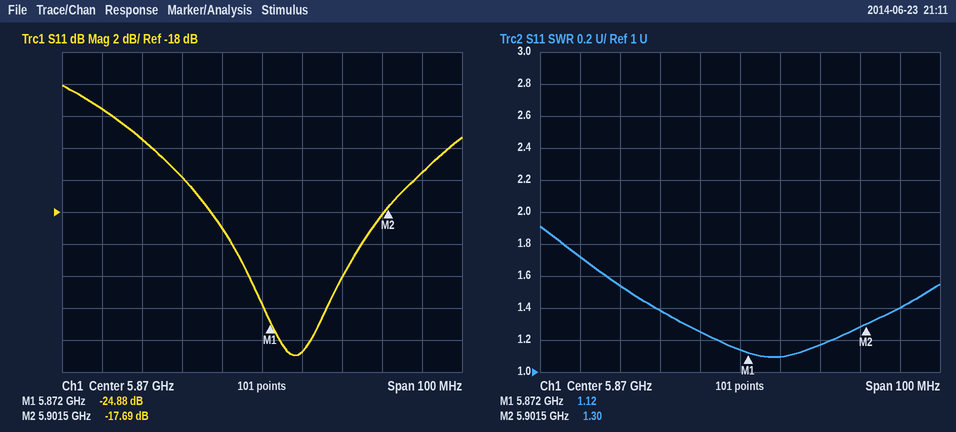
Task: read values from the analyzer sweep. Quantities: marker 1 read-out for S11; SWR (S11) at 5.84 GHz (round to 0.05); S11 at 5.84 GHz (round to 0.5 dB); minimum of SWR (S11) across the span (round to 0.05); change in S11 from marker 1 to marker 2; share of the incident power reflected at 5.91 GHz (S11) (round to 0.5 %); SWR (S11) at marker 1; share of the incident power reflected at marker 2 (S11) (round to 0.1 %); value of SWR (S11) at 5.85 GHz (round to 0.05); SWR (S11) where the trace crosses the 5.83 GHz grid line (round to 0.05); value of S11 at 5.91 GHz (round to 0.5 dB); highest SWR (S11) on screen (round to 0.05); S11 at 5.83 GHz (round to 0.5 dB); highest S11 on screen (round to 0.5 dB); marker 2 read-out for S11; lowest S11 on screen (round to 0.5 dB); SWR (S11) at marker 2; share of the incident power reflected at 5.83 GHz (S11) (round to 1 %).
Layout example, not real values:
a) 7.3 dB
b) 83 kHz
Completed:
a) -24.88 dB
b) 1.55
c) -13.5 dB
d) 1.10
e) 7.19 dB
f) 3.0 %
g) 1.12
h) 1.7 %
i) 1.40
j) 1.70
k) -15.5 dB
l) 1.90
m) -11.5 dB
n) -10.0 dB
o) -17.69 dB
p) -27.0 dB
q) 1.30
r) 7 %
